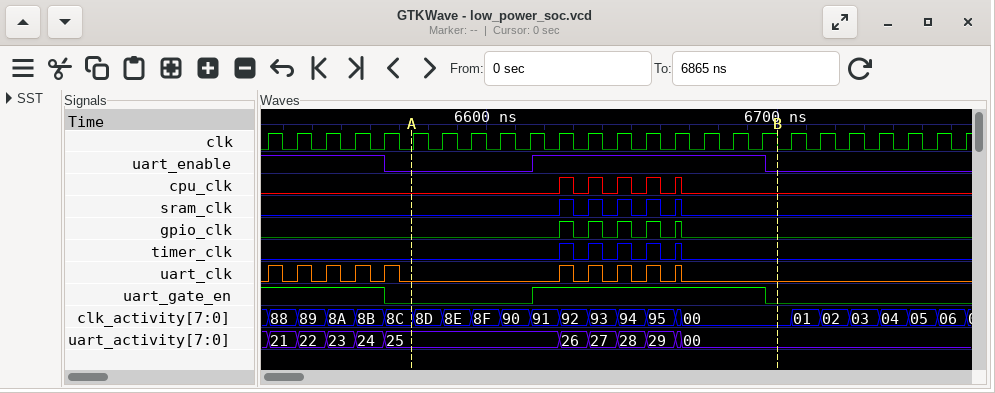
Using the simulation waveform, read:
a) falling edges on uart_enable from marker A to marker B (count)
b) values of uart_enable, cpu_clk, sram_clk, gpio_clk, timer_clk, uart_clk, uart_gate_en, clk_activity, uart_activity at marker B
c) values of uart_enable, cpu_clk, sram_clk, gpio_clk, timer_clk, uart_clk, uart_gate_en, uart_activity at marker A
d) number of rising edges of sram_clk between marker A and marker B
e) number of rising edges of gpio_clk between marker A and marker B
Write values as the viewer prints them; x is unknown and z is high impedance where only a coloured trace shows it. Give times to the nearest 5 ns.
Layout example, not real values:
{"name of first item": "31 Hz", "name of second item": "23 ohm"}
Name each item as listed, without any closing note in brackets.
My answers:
{"falling edges on uart_enable from marker A to marker B": "1", "values of uart_enable, cpu_clk, sram_clk, gpio_clk, timer_clk, uart_clk, uart_gate_en, clk_activity, uart_activity at marker B": "uart_enable=0, cpu_clk=0, sram_clk=0, gpio_clk=0, timer_clk=0, uart_clk=0, uart_gate_en=0, clk_activity=00, uart_activity=00", "values of uart_enable, cpu_clk, sram_clk, gpio_clk, timer_clk, uart_clk, uart_gate_en, uart_activity at marker A": "uart_enable=0, cpu_clk=0, sram_clk=0, gpio_clk=0, timer_clk=0, uart_clk=0, uart_gate_en=0, uart_activity=25", "number of rising edges of sram_clk between marker A and marker B": "5", "number of rising edges of gpio_clk between marker A and marker B": "5"}
